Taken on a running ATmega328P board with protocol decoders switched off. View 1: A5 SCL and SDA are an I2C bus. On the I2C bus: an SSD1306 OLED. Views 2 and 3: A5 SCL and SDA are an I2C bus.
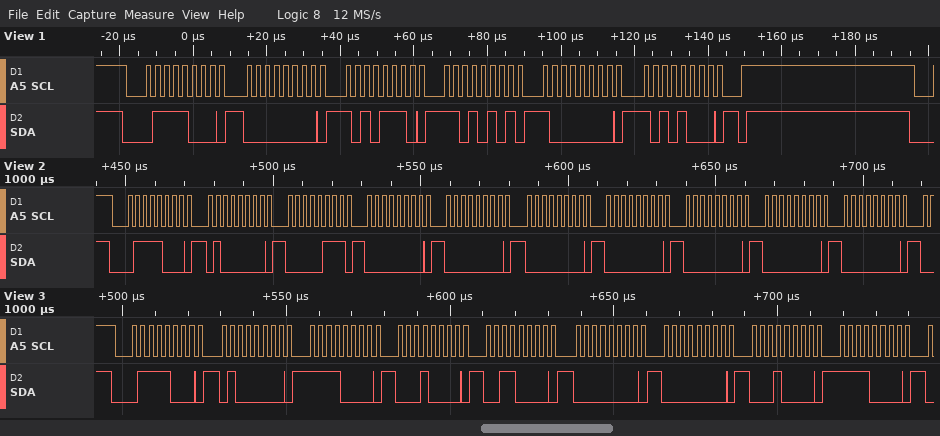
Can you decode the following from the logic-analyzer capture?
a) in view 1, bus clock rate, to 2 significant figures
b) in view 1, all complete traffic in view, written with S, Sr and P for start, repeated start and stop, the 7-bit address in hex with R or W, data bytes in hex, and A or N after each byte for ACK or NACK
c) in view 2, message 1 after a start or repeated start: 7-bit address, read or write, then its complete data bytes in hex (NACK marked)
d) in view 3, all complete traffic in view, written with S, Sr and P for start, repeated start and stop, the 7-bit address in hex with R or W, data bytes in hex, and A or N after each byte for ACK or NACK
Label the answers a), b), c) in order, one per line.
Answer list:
a) 400 kHz
b) S 3CW A 00 A AE A D5 A 80 A A8 A P
c) 0x3C write: 40 07 00 00 00 00 00 00 00
d) S 3CW A 40 A F0 A 10 A 30 A 00 A 00 A 10 A F0 A
